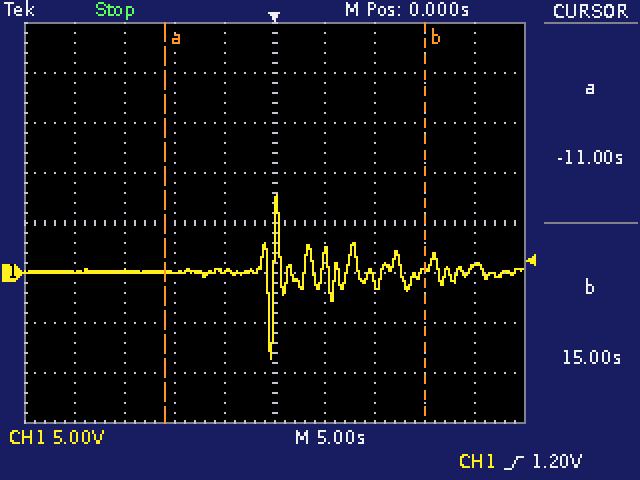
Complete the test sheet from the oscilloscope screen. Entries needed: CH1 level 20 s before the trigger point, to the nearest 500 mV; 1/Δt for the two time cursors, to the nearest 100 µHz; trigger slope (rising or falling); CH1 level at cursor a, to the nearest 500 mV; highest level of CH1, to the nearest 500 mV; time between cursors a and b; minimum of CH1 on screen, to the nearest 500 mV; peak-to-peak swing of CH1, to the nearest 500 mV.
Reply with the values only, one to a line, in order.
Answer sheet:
0.0 V
38.5 mHz
rising
0.0 V
8.0 V
26.0 s
-8.5 V
16.5 V
